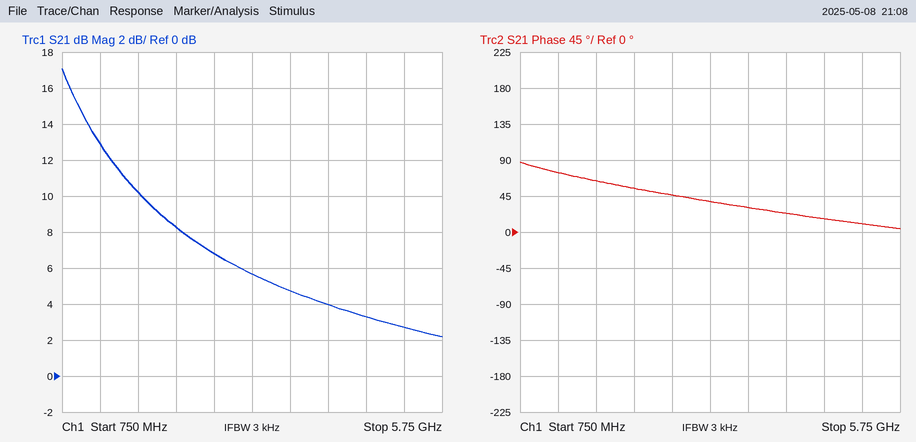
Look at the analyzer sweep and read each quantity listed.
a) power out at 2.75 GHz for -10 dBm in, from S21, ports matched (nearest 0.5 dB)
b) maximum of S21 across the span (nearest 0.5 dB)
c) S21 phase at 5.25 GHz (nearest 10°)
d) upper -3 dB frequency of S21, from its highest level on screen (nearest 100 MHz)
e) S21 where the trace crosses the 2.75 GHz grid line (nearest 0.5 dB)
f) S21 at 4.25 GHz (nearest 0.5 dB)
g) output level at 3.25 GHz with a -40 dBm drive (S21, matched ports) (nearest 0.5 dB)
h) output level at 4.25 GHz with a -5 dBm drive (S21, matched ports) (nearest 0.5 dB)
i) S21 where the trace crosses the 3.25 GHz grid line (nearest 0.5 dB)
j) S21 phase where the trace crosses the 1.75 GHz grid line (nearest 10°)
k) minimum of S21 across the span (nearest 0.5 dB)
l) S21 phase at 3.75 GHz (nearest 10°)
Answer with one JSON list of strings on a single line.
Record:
["-3.0 dBm", "17.0 dB", "10°", "1.1 GHz", "7.0 dB", "4.0 dB", "-34.5 dBm", "-1.0 dBm", "5.5 dB", "60°", "2.0 dB", "30°"]
